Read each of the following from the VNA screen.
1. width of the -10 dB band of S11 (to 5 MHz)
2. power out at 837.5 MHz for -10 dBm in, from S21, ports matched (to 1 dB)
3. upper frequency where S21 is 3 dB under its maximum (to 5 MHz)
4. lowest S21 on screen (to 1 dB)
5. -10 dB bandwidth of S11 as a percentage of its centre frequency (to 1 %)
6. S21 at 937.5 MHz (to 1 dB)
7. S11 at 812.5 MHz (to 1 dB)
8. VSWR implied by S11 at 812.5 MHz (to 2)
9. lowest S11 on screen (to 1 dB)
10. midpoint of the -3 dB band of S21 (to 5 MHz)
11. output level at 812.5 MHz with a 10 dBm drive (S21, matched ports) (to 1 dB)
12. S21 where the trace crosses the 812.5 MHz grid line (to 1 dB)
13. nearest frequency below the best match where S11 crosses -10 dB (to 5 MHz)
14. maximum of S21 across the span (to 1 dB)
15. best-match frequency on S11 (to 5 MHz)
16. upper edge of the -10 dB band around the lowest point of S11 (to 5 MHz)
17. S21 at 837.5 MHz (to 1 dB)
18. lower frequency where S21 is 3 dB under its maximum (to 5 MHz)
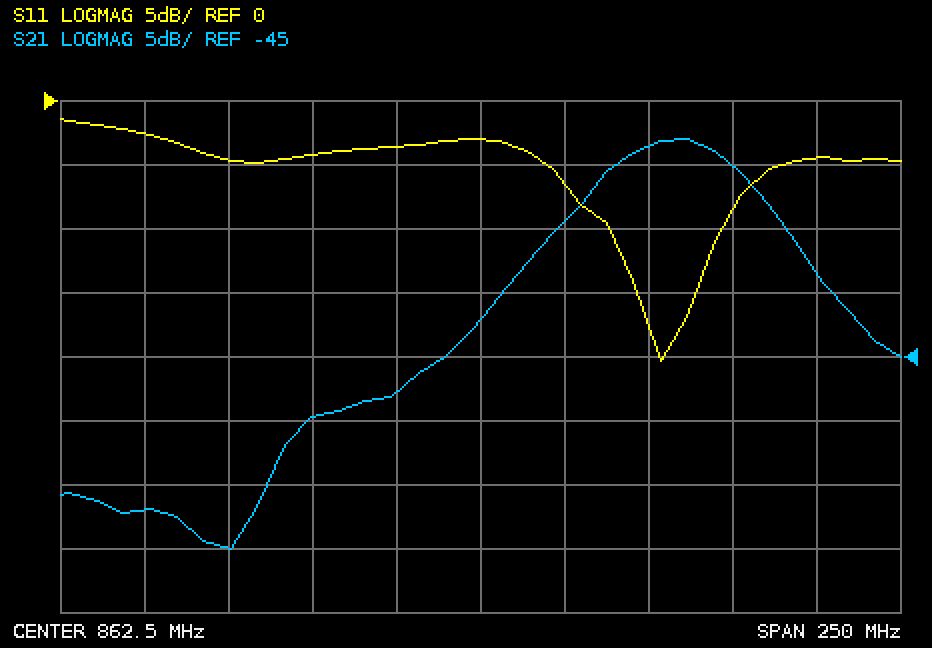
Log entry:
35 MHz
-58 dBm
940 MHz
-60 dB
4 %
-30 dB
-4 dB
4
-20 dB
920 MHz
-40 dBm
-50 dB
900 MHz
-28 dB
915 MHz
935 MHz
-48 dB
900 MHz
